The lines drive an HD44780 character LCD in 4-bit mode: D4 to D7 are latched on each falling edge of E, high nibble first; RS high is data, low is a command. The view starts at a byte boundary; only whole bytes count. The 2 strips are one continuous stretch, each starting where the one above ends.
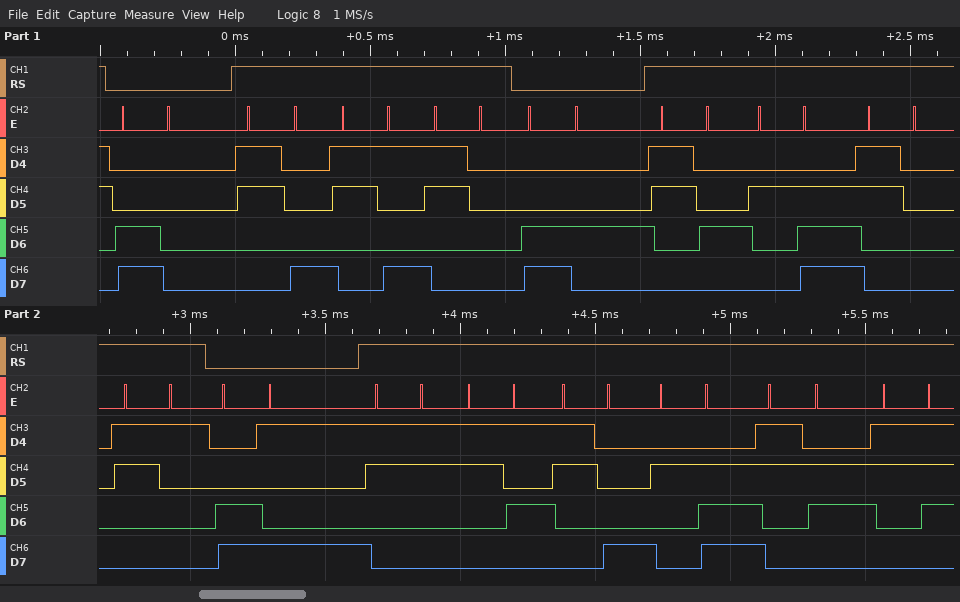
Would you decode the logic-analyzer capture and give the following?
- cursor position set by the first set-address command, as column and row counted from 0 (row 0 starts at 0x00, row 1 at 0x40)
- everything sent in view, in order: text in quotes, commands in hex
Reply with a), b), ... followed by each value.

a) column 0, row 1
b) 0xC0 "890" 0xC4 "4.01" 0xC9 "358.67"
